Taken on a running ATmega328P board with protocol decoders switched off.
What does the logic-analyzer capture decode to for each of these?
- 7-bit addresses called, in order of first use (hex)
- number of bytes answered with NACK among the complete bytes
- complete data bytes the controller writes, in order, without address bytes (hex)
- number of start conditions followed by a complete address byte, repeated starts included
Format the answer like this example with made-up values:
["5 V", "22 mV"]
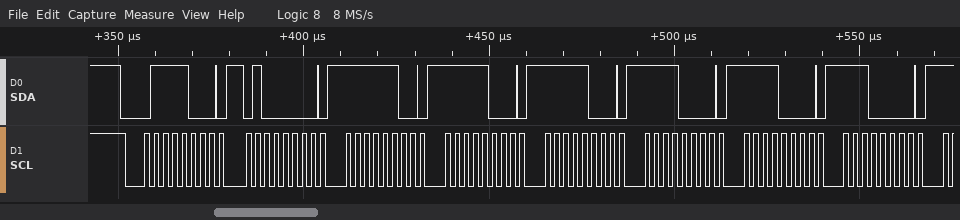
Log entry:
["0x3C", "0", "40 FC F8 F8 F0 F0 E0", "1"]
